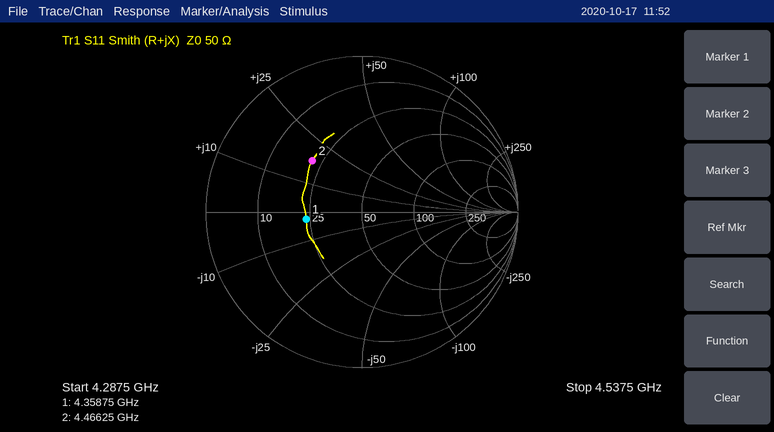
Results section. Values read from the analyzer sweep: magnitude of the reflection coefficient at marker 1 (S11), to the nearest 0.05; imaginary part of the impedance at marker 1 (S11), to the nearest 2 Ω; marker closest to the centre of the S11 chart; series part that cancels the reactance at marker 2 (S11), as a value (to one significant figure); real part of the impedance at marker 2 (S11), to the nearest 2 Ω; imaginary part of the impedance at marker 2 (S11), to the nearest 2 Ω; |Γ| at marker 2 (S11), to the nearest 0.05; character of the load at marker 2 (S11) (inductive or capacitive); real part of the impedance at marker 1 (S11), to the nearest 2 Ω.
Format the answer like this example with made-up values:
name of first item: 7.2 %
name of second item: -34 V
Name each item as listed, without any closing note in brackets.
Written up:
magnitude of the reflection coefficient at marker 1 (S11), to the nearest 0.05: 0.35
imaginary part of the impedance at marker 1 (S11), to the nearest 2 Ω: -2 Ω
marker closest to the centre of the S11 chart: marker 1
series part that cancels the reactance at marker 2 (S11), as a value: 2 pF
real part of the impedance at marker 2 (S11), to the nearest 2 Ω: 22 Ω
imaginary part of the impedance at marker 2 (S11), to the nearest 2 Ω: +18 Ω
|Γ| at marker 2 (S11), to the nearest 0.05: 0.45
character of the load at marker 2 (S11): inductive
real part of the impedance at marker 1 (S11), to the nearest 2 Ω: 24 Ω
